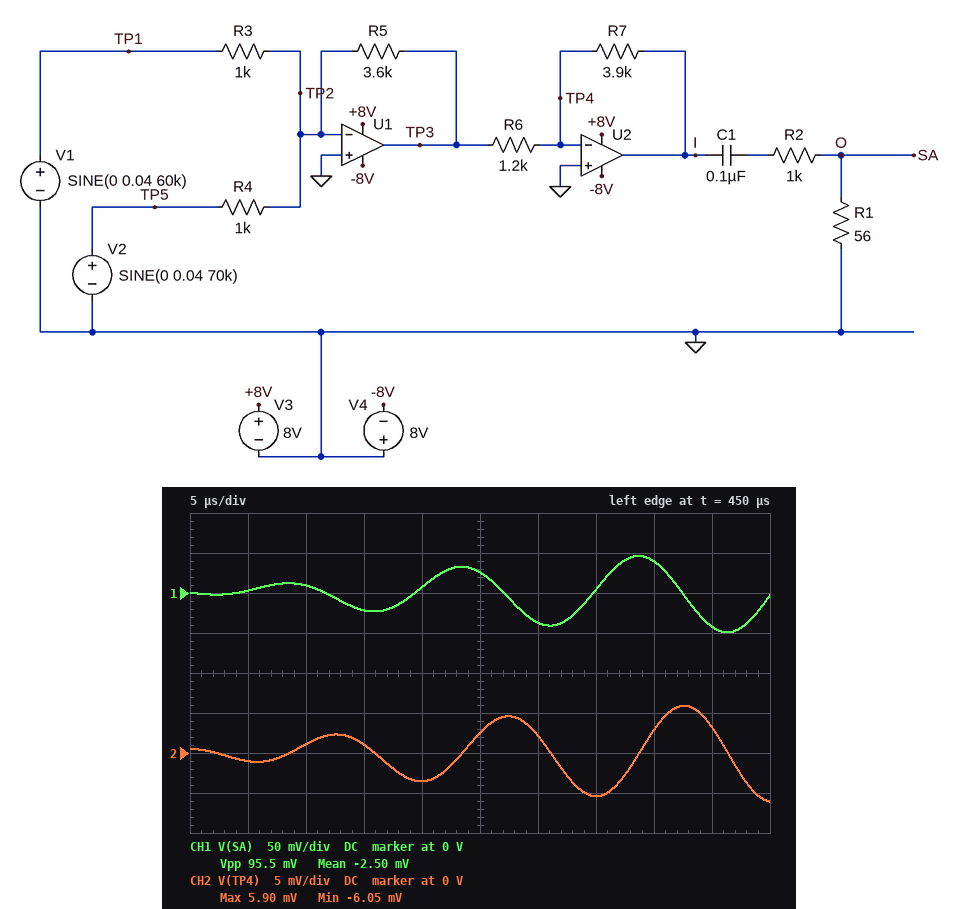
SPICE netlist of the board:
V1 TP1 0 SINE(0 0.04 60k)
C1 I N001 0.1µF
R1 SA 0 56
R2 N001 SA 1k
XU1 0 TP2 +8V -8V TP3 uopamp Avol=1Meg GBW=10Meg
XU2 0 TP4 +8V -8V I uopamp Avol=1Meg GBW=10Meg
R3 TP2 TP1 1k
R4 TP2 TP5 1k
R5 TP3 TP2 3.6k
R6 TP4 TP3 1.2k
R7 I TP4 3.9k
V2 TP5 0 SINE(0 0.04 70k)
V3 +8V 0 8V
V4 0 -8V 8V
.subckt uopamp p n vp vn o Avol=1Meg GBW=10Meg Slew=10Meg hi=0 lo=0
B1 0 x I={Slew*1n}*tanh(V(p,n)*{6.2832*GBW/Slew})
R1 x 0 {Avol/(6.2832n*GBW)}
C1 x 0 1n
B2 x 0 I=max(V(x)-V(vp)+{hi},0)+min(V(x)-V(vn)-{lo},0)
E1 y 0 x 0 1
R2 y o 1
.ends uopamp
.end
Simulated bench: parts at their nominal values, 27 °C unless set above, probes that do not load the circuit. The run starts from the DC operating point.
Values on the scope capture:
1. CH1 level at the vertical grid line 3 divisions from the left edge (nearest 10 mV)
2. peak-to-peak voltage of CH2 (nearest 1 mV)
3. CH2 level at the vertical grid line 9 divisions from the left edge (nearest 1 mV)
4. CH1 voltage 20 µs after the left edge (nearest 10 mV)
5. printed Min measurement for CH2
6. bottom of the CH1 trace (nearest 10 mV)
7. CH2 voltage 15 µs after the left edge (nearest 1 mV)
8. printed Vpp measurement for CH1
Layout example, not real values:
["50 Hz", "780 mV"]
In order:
["-20 mV", "12 mV", "3 mV", "10 mV", "-6.05 mV", "-50 mV", "1 mV", "95.5 mV"]
